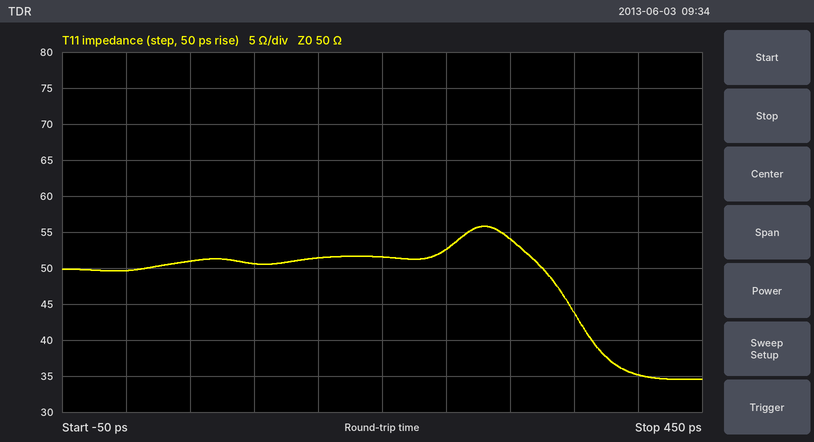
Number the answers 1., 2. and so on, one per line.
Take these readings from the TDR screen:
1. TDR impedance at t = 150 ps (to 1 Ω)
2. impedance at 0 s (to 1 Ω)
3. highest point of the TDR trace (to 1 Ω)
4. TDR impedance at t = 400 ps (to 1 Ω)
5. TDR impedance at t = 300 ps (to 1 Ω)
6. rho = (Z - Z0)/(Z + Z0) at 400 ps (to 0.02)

1. 51 Ω
2. 50 Ω
3. 56 Ω
4. 35 Ω
5. 54 Ω
6. -0.18
